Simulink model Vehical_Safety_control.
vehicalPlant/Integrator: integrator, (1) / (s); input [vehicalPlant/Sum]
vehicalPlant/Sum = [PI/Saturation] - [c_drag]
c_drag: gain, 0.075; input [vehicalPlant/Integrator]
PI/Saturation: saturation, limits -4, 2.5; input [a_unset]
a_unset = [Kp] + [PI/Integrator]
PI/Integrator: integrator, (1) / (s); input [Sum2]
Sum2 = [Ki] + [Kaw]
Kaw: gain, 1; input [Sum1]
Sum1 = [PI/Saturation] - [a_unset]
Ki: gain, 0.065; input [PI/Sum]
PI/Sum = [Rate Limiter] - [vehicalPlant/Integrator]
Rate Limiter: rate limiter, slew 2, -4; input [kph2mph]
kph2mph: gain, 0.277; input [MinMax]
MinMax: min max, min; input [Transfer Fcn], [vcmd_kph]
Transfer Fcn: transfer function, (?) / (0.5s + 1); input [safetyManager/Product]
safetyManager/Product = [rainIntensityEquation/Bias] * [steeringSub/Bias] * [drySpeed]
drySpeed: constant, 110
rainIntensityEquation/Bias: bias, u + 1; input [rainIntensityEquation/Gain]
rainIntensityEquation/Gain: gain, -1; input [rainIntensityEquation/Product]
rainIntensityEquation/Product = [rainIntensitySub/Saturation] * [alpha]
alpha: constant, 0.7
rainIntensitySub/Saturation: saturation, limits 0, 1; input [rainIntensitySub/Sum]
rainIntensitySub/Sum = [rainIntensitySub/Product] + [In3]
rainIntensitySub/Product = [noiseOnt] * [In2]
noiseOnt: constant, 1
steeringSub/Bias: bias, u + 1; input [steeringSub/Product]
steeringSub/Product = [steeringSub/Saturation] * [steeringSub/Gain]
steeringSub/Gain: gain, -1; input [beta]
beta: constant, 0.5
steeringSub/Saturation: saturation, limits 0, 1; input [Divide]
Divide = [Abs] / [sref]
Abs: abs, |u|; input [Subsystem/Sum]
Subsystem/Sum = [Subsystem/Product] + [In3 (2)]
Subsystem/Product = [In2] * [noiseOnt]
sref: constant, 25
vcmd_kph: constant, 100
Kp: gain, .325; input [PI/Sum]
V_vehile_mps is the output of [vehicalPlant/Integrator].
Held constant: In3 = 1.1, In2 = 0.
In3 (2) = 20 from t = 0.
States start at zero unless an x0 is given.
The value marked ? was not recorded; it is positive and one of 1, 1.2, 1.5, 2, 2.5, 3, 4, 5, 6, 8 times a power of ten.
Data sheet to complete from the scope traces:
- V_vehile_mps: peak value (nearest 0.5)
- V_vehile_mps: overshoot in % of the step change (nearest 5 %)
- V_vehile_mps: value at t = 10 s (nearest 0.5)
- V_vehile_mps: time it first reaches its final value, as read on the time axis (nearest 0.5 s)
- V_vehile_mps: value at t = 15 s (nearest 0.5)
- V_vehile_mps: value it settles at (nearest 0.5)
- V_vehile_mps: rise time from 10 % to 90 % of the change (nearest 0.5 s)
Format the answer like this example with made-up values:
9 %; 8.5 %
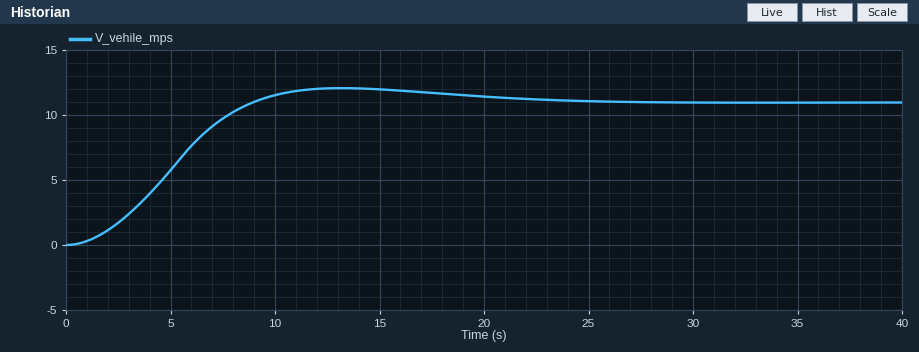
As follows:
12.0; 10 %; 11.5; 9.0 s; 12.0; 11.0; 5.5 s
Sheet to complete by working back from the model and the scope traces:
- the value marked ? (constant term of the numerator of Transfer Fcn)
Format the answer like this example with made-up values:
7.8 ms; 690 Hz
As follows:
2
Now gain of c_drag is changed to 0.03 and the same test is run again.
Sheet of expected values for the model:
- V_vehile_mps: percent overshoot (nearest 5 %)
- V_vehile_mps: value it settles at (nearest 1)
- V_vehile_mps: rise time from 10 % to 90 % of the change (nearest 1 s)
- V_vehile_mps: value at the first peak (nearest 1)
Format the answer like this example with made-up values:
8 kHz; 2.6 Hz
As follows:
15 %; 11; 5 s; 13
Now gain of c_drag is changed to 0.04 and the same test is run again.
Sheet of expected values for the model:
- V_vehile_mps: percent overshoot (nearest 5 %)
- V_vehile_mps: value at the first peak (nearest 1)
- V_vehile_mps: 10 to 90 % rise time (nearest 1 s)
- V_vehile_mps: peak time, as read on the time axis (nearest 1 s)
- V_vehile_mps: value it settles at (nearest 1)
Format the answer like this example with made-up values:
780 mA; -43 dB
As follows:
15 %; 13; 5 s; 13 s; 11
